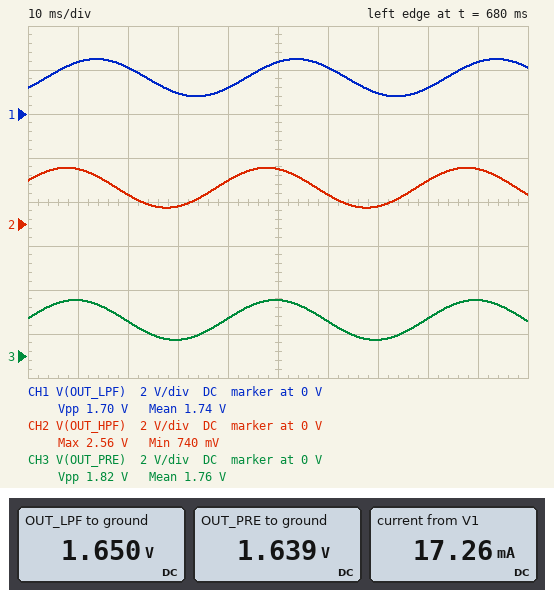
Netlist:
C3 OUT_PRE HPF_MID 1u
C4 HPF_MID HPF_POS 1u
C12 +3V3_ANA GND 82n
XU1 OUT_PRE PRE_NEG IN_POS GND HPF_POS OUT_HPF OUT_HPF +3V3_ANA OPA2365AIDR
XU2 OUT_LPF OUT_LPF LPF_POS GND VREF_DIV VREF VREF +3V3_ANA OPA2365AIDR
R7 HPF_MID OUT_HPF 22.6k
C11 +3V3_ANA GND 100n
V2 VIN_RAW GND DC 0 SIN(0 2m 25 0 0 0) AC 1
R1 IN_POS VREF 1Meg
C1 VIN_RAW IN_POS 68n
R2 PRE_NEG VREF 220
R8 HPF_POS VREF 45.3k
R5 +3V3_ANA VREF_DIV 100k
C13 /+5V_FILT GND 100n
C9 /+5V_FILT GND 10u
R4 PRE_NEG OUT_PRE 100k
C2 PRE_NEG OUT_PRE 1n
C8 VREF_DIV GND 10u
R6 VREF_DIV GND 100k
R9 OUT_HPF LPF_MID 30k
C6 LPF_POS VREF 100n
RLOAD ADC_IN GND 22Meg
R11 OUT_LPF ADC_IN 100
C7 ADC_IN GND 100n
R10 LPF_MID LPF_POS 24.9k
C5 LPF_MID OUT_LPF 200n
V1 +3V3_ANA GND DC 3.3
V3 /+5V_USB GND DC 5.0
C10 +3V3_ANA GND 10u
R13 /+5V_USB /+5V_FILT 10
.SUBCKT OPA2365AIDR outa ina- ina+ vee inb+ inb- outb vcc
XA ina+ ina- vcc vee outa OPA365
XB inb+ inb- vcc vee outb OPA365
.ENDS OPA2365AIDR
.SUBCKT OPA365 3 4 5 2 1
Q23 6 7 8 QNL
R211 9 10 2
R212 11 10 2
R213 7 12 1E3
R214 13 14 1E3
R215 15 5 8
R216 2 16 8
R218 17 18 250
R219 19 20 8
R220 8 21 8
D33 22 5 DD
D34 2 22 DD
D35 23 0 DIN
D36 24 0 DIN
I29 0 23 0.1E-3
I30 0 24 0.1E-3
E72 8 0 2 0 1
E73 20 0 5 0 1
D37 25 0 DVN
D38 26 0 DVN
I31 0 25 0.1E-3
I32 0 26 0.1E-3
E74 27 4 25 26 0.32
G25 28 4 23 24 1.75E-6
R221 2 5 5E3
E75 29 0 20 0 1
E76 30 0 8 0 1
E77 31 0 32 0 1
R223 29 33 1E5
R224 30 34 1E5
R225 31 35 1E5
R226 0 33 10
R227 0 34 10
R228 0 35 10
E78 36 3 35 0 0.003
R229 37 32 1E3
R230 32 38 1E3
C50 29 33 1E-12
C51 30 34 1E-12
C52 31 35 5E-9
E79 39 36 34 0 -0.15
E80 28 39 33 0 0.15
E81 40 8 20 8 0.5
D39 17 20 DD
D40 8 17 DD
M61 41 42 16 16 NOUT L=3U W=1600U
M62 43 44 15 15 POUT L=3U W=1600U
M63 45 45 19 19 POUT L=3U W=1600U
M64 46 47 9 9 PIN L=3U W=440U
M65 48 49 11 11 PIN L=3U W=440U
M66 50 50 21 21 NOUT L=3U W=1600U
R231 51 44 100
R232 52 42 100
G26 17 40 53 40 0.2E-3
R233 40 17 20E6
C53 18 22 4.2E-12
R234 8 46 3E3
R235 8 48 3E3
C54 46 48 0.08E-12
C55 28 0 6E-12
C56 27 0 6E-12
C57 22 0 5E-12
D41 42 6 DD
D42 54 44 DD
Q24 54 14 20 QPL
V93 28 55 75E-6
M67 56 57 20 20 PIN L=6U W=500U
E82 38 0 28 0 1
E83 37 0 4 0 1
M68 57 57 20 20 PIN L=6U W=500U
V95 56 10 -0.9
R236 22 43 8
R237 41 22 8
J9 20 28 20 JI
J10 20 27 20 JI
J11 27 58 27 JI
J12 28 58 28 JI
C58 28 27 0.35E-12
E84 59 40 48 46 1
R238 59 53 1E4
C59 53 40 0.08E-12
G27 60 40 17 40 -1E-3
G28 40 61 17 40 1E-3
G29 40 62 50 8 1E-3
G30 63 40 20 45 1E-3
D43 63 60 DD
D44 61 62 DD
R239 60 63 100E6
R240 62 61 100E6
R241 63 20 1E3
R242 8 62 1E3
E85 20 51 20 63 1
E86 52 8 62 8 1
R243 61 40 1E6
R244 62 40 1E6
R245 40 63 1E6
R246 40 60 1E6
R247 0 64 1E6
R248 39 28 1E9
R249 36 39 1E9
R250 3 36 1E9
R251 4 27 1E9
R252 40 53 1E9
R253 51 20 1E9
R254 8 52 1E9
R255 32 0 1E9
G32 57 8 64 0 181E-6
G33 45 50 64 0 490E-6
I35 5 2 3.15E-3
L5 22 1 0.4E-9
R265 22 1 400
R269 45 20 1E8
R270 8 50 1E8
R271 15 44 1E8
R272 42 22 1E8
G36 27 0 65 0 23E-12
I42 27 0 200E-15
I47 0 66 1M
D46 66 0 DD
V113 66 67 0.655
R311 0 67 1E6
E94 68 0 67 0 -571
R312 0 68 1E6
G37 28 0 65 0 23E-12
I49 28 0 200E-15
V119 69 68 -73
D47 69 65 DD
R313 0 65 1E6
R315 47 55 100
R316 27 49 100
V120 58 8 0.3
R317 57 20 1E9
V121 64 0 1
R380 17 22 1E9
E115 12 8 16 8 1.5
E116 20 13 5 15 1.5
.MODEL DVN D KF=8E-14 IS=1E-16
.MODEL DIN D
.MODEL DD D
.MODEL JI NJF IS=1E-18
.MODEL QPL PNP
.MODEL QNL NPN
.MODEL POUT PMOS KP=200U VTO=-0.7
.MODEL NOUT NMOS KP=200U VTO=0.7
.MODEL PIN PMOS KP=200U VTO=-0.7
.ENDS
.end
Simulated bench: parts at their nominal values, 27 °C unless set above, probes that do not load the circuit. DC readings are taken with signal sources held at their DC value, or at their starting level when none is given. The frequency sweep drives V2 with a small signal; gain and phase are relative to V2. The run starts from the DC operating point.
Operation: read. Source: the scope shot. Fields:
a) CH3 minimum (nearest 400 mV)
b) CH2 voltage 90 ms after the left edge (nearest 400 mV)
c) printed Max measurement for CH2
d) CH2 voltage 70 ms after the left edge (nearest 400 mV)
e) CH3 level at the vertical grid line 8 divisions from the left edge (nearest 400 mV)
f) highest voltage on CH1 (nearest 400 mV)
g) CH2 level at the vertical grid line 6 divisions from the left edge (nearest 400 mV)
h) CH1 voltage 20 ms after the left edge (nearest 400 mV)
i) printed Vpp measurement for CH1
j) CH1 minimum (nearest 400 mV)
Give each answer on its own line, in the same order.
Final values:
800 mV
2.4 V
2.56 V
800 mV
1.6 V
2.4 V
1.2 V
2.0 V
1.70 V
800 mV
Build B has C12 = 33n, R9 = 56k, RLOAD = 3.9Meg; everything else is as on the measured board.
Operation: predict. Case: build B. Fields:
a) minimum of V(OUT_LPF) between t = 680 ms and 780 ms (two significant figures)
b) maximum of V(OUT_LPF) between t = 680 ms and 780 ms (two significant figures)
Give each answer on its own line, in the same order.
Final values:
960 mV
2.3 V
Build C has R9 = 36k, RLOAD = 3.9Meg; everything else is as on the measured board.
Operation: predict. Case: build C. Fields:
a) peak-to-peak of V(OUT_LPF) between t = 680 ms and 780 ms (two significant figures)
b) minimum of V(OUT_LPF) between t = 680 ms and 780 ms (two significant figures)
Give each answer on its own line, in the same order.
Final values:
1.6 V
830 mV
